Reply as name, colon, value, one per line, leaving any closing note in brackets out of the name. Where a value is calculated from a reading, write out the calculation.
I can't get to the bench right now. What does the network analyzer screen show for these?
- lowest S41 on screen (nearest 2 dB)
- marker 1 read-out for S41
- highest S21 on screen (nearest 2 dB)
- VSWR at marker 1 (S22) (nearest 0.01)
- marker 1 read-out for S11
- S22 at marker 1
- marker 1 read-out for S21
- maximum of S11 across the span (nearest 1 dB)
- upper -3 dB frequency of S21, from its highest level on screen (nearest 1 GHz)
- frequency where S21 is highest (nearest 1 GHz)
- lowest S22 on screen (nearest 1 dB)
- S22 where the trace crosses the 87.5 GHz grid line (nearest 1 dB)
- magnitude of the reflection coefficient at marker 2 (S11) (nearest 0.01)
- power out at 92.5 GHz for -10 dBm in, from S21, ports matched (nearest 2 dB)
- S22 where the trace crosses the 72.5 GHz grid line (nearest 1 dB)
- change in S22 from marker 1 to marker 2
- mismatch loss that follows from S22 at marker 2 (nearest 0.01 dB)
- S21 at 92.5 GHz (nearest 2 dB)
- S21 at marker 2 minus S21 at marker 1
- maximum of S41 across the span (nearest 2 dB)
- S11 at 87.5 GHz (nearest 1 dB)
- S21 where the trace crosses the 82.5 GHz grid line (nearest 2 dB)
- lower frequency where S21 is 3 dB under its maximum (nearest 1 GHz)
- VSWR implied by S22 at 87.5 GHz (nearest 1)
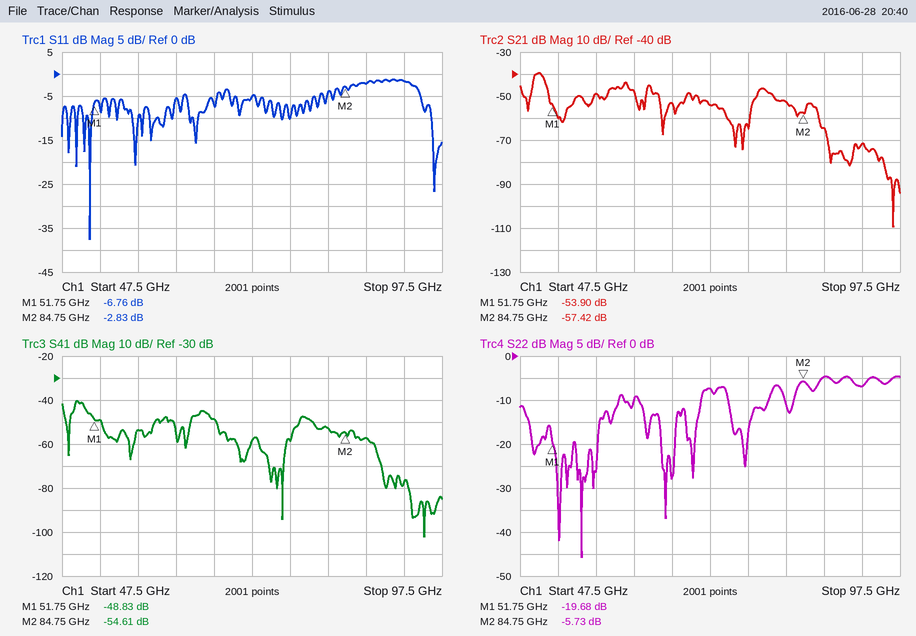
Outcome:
lowest S41 on screen: -102 dB
marker 1 read-out for S41: -48.83 dB
highest S21 on screen: -40 dB
VSWR at marker 1 (S22): (1 + 0.1038)/(1 − 0.1038) ≈ 1.23
marker 1 read-out for S11: -6.76 dB
S22 at marker 1: -19.68 dB
marker 1 read-out for S21: -53.90 dB
maximum of S11 across the span: -1 dB
upper -3 dB frequency of S21, from its highest level on screen: 51 GHz
frequency where S21 is highest: 50 GHz
lowest S22 on screen: -46 dB
S22 where the trace crosses the 87.5 GHz grid line: -5 dB
magnitude of the reflection coefficient at marker 2 (S11): 10^(-2.83/20) ≈ 0.72
power out at 92.5 GHz for -10 dBm in, from S21, ports matched: -10 dBm + (-72 dB) = -82 dBm
S22 where the trace crosses the 72.5 GHz grid line: -7 dB
change in S22 from marker 1 to marker 2: -5.73 − (-19.68) = 13.95 dB
mismatch loss that follows from S22 at marker 2: −10 log10(1 − 10^(-5.73/10)) ≈ 1.35 dB
S21 at 92.5 GHz: -72 dB
S21 at marker 2 minus S21 at marker 1: -57.42 − (-53.9) = -3.52 dB
maximum of S41 across the span: -40 dB
S11 at 87.5 GHz: -2 dB
S21 where the trace crosses the 82.5 GHz grid line: -52 dB
lower frequency where S21 is 3 dB under its maximum: 49 GHz
VSWR implied by S22 at 87.5 GHz: |Γ| = 10^(-5/20) = 0.5623; VSWR = (1 + 0.5623)/(1 − 0.5623) ≈ 4
